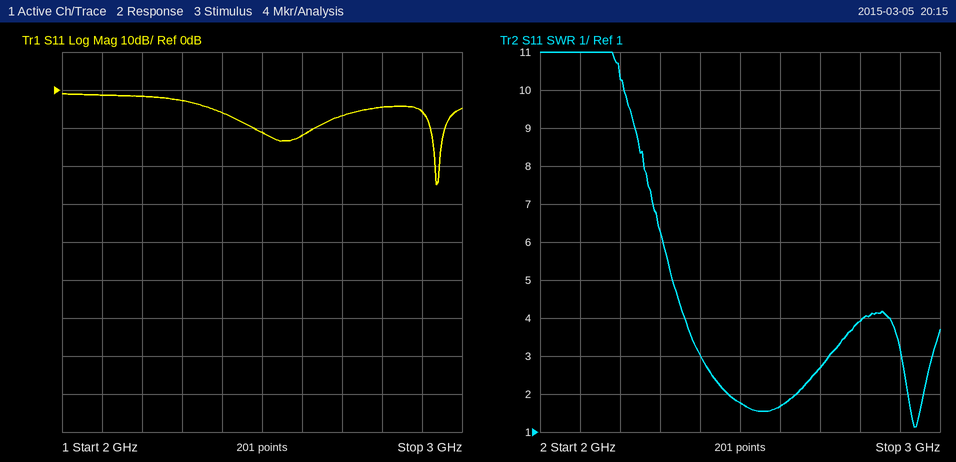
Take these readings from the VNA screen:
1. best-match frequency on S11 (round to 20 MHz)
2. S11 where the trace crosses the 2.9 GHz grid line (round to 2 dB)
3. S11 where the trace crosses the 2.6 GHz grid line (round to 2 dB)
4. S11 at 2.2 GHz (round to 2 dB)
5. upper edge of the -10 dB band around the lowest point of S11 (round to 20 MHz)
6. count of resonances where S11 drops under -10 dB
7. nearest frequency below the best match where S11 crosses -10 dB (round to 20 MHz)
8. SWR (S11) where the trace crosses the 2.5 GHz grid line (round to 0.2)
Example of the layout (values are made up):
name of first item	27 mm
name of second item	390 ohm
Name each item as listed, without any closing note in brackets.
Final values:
best-match frequency on S11	2.94 GHz
S11 where the trace crosses the 2.9 GHz grid line	-6 dB
S11 where the trace crosses the 2.6 GHz grid line	-12 dB
S11 at 2.2 GHz	-2 dB
upper edge of the -10 dB band around the lowest point of S11	2.96 GHz
count of resonances where S11 drops under -10 dB	2
nearest frequency below the best match where S11 crosses -10 dB	2.92 GHz
SWR (S11) where the trace crosses the 2.5 GHz grid line	1.8
